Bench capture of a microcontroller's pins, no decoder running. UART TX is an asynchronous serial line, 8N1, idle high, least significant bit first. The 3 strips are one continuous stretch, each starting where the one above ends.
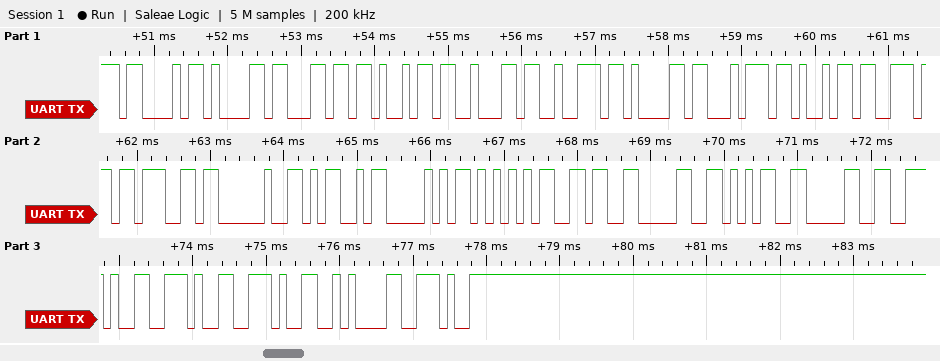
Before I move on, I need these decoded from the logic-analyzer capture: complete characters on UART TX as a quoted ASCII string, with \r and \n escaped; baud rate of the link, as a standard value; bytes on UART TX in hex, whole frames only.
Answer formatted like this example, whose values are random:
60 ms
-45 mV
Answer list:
"Calibrating MPU6050...\n."
9600 baud
43 61 6C 69 62 72 61 74 69 6E 67 20 4D 50 55 36 30 35 30 2E 2E 2E 0A 2E
